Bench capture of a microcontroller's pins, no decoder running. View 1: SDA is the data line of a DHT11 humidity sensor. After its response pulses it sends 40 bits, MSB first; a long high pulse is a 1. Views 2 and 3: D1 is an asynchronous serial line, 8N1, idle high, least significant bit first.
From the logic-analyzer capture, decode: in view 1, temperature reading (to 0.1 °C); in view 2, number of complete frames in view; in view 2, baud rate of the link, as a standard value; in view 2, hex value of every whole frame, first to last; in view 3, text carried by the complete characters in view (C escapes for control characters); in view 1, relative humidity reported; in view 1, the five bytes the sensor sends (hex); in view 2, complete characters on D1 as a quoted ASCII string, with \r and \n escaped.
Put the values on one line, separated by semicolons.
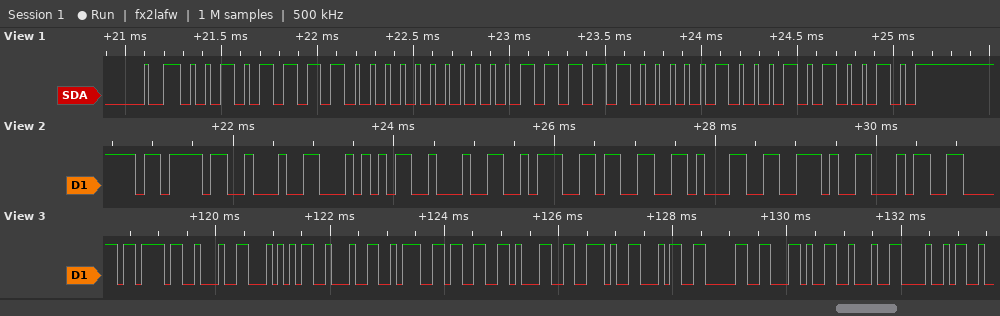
31.4 °C; 9; 9600 baud; 7B 22 54 22 3A 33 31 2E 34; "{\"T\":31.40,\"H"; 47 %; 2F 00 1F 04 52; "{\"T\":31.4"
